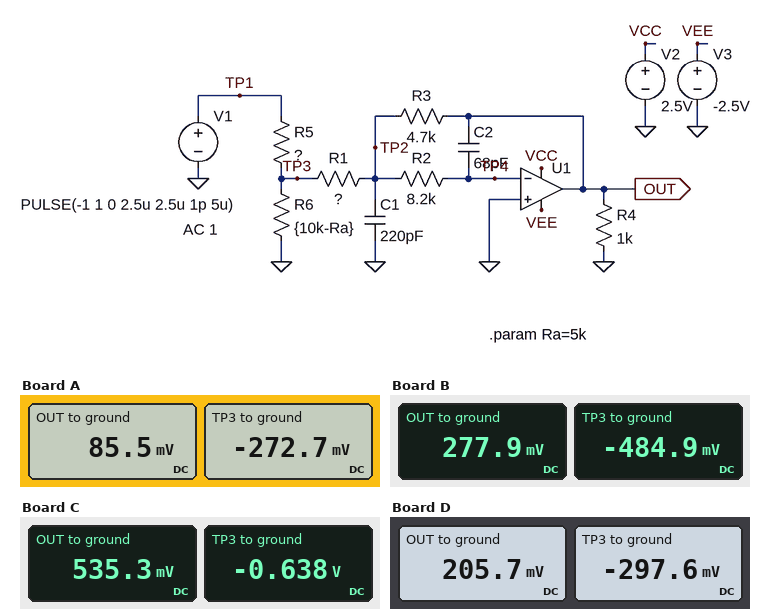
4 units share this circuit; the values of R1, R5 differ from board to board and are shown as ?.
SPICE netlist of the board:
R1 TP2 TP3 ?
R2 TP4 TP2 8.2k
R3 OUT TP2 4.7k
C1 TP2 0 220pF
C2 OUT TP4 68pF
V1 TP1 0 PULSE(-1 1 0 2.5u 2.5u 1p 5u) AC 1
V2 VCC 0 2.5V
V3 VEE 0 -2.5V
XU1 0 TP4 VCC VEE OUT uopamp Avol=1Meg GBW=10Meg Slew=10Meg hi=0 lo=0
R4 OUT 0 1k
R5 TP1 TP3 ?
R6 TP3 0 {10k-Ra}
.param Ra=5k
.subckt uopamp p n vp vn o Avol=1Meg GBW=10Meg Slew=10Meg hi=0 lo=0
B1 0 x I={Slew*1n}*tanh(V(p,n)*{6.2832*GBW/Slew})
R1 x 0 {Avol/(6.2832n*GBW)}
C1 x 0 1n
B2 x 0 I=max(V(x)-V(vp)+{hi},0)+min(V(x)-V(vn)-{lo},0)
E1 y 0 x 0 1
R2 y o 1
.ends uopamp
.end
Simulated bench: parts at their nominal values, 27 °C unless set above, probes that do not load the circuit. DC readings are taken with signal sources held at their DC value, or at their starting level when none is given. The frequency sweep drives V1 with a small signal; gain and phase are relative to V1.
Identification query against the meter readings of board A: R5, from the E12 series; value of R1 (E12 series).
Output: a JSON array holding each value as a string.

["10 kΩ", "15 kΩ"]
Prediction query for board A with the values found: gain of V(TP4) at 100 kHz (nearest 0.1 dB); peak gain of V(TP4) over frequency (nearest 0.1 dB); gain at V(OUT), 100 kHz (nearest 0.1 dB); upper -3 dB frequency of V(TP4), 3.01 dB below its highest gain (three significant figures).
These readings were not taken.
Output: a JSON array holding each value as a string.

["-61.4 dB", "-57.5 dB", "-21.4 dB", "385 kHz"]
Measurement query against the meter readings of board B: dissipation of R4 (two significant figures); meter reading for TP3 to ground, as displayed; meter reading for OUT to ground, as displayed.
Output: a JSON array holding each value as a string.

["77 µW", "-484.9 mV", "277.9 mV"]
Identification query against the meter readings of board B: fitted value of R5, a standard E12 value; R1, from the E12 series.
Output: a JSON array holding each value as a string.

["3.3 kΩ", "8.2 kΩ"]
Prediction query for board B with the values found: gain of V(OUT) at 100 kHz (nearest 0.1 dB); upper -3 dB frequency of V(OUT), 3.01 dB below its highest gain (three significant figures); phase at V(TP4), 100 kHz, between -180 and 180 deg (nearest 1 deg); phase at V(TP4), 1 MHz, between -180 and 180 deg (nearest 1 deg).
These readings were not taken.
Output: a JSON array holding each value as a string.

["-11.5 dB", "197 kHz", "46 deg", "-78 deg"]
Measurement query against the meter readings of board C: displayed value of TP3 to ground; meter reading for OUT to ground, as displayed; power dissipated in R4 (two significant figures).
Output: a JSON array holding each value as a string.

["-0.638 V", "535.3 mV", "290 µW"]
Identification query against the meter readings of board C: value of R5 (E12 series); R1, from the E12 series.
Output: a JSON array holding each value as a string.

["1.5 kΩ", "5.6 kΩ"]
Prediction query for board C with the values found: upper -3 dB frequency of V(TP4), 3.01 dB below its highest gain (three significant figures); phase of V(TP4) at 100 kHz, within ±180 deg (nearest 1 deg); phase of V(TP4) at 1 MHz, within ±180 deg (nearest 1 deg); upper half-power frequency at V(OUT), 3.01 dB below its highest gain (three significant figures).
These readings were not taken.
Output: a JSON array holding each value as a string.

["439 kHz", "43 deg", "-76 deg", "172 kHz"]
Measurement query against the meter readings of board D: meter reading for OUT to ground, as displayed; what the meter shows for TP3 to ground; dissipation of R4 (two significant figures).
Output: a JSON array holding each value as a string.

["205.7 mV", "-297.6 mV", "42 µW"]
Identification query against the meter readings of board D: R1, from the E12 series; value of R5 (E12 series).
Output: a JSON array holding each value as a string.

["6.8 kΩ", "6.8 kΩ"]
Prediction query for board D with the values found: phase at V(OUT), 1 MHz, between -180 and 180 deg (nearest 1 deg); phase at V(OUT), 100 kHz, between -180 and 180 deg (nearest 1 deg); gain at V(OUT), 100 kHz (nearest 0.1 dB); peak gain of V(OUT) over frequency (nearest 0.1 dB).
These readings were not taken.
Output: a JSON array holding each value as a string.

["12 deg", "136 deg", "-14.2 dB", "-13.7 dB"]
